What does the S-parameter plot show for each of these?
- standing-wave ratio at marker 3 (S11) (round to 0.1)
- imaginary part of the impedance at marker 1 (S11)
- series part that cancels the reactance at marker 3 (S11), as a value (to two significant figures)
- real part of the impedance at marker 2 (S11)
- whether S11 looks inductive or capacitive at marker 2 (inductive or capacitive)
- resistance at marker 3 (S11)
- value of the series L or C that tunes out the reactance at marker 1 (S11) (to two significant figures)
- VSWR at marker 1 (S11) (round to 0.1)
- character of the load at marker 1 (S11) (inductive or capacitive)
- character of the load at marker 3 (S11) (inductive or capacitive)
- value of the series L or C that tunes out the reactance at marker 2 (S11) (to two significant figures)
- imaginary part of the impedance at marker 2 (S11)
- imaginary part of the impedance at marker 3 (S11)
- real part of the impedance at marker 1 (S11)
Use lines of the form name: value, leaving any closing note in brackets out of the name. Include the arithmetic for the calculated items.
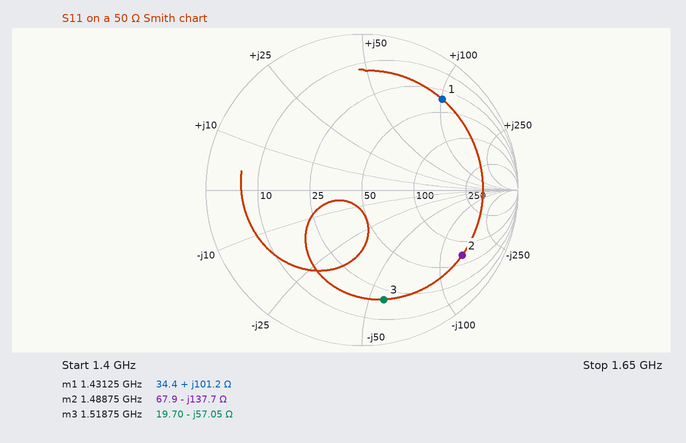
standing-wave ratio at marker 3 (S11): 6.1
imaginary part of the impedance at marker 1: +101.2 Ω
series part that cancels the reactance at marker 3 (S11), as a value: L = 57.05 Ω/(2π × 1.51875 GHz) ≈ 6.0 nH
real part of the impedance at marker 2: 67.9 Ω
whether S11 looks inductive or capacitive at marker 2: capacitive
resistance at marker 3: 19.70 Ω
value of the series L or C that tunes out the reactance at marker 1 (S11): C = 1/(2π × 1.43125 GHz × 101.2 Ω) ≈ 1.1 pF
VSWR at marker 1 (S11): 8.0
character of the load at marker 1 (S11): inductive
character of the load at marker 3 (S11): capacitive
value of the series L or C that tunes out the reactance at marker 2 (S11): L = 137.7 Ω/(2π × 1.48875 GHz) ≈ 15 nH
imaginary part of the impedance at marker 2: -137.7 Ω
imaginary part of the impedance at marker 3: -57.05 Ω
real part of the impedance at marker 1: 34.4 Ω
